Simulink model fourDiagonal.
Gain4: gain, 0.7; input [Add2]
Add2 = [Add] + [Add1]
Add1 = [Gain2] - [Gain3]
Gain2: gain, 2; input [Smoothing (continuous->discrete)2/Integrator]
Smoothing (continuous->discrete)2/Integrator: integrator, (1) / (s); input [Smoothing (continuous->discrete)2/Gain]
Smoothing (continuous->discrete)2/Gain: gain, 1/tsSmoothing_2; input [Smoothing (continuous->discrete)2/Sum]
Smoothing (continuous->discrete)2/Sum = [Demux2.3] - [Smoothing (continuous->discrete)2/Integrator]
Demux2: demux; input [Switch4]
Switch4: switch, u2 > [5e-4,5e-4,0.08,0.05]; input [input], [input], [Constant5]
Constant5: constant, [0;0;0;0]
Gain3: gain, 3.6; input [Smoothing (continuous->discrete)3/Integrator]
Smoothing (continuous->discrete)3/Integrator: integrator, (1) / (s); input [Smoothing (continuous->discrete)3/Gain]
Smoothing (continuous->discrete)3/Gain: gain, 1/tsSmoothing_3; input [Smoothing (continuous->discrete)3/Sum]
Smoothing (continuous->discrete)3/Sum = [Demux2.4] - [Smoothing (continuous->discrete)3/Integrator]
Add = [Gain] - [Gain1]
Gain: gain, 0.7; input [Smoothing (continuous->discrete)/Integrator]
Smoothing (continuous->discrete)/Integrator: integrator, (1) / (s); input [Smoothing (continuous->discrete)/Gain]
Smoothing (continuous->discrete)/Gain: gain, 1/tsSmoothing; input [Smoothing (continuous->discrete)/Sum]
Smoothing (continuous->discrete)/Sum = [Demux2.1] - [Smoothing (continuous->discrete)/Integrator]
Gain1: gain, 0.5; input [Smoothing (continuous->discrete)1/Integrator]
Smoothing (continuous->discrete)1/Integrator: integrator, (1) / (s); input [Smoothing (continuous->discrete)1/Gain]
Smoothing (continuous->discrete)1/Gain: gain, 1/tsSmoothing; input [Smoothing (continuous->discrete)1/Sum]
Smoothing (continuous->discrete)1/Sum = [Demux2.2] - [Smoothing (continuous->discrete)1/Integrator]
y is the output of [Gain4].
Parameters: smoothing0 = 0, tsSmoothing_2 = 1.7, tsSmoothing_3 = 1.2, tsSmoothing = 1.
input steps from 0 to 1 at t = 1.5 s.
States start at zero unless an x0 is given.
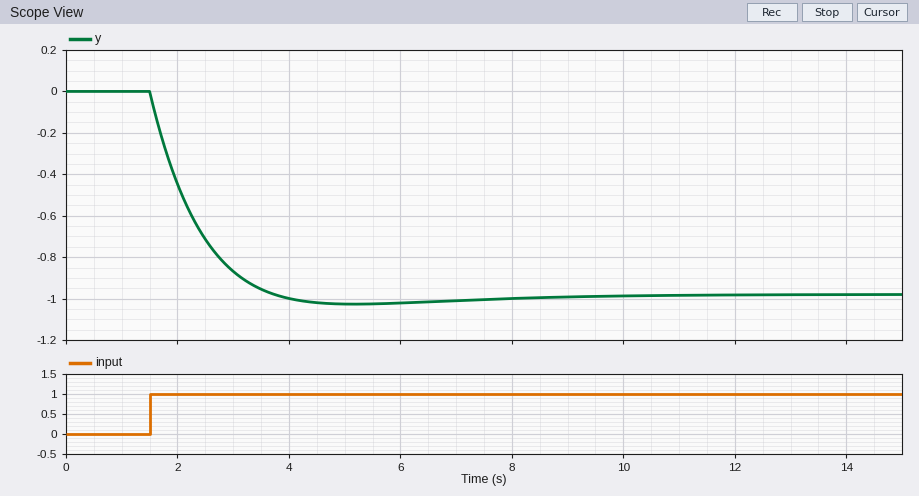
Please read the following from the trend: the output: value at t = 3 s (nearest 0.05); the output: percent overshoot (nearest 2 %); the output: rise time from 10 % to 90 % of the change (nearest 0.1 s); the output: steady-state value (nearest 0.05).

-0.85
4 %
1.5 s
-1.00
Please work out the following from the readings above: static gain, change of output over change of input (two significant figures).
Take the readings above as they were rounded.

-1.0
